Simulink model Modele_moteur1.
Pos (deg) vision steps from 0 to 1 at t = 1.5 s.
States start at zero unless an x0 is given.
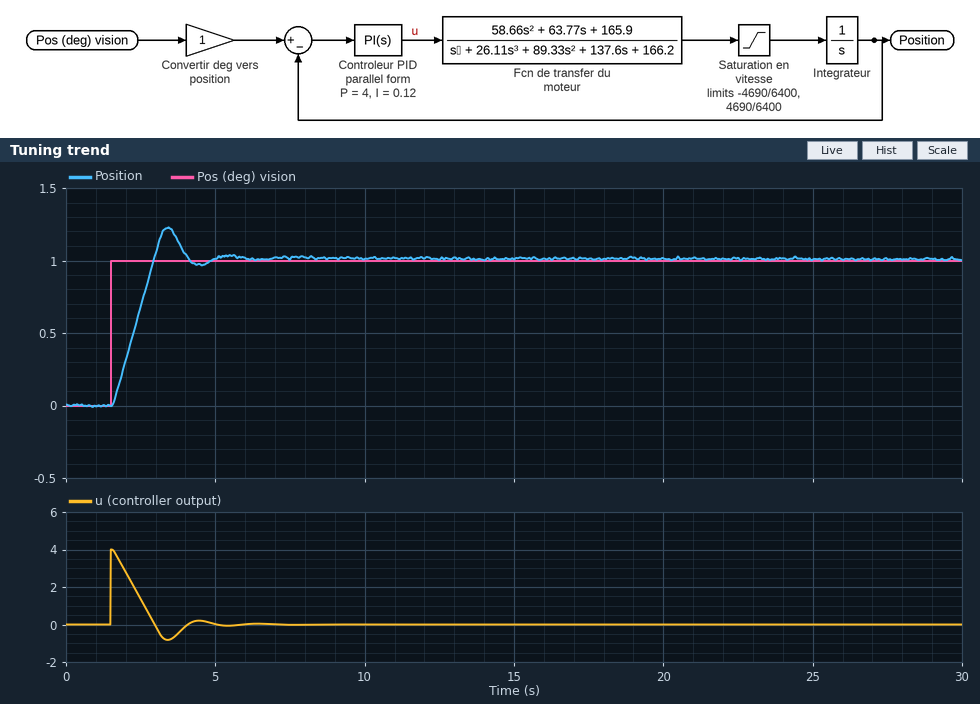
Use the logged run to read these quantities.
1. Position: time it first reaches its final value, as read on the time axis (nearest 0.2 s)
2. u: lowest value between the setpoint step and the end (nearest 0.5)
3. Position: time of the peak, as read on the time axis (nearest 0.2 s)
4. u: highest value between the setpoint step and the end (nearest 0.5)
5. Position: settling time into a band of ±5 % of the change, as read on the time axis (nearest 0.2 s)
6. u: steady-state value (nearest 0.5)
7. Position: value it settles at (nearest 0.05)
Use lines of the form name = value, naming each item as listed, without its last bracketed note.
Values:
Position: time it first reaches its final value, as read on the time axis = 3.0 s
u: lowest value between the setpoint step and the end = -1.0
Position: time of the peak, as read on the time axis = 3.4 s
u: highest value between the setpoint step and the end = 4.0
Position: settling time into a band of ±5 % of the change, as read on the time axis = 4.0 s
u: steady-state value = 0.0
Position: value it settles at = 1.00
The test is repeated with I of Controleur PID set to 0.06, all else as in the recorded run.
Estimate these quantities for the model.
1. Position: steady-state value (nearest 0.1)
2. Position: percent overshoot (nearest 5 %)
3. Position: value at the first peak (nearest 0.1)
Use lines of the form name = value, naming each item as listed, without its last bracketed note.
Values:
Position: steady-state value = 1.0
Position: percent overshoot = 20 %
Position: value at the first peak = 1.2
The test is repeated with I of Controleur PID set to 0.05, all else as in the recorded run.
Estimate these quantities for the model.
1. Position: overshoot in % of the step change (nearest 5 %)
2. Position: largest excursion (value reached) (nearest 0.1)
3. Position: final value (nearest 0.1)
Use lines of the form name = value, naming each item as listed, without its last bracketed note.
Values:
Position: overshoot in % of the step change = 20 %
Position: largest excursion (value reached) = 1.2
Position: final value = 1.0
